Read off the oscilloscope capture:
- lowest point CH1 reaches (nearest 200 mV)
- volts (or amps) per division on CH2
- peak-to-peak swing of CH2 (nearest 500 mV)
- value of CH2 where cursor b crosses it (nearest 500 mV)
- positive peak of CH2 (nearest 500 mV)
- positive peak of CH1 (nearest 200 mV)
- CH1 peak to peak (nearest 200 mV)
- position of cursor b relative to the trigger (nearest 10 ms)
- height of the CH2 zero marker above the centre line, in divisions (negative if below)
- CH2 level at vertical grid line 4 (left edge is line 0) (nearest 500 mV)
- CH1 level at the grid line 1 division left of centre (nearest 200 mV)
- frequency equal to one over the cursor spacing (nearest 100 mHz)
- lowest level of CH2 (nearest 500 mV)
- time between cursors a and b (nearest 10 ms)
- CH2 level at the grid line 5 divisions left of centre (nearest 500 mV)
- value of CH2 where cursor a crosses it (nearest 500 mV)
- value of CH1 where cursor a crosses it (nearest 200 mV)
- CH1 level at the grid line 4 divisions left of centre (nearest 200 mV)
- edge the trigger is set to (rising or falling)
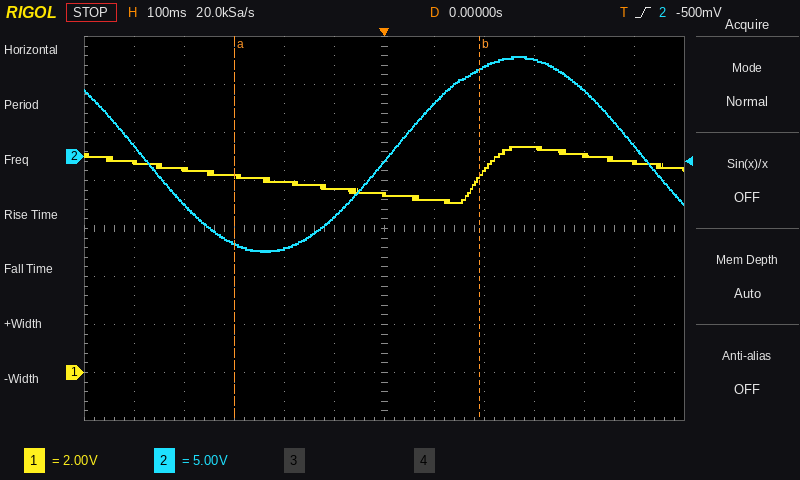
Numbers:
7.0 V
5 V
20.5 V
9.0 V
10.5 V
9.4 V
2.4 V
+190 ms
+1.5 div
-9.5 V
7.6 V
2.0 Hz
-10.0 V
490 ms
1.0 V
-9.0 V
8.2 V
8.4 V
rising
